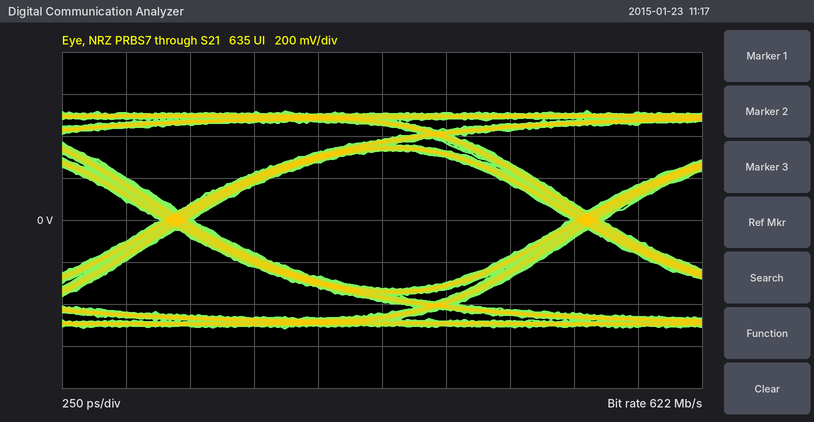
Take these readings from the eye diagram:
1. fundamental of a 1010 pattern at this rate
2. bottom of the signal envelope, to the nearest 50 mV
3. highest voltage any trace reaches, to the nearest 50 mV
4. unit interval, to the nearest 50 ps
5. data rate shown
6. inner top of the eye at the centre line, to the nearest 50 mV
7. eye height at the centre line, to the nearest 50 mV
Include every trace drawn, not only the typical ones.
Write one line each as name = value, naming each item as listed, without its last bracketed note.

fundamental of a 1010 pattern at this rate = 311 MHz
bottom of the signal envelope, to the nearest 50 mV = -500 mV
highest voltage any trace reaches, to the nearest 50 mV = 500 mV
unit interval, to the nearest 50 ps = 1.60 ns
data rate shown = 622 Mb/s
inner top of the eye at the centre line, to the nearest 50 mV = 350 mV
eye height at the centre line, to the nearest 50 mV = 650 mV
